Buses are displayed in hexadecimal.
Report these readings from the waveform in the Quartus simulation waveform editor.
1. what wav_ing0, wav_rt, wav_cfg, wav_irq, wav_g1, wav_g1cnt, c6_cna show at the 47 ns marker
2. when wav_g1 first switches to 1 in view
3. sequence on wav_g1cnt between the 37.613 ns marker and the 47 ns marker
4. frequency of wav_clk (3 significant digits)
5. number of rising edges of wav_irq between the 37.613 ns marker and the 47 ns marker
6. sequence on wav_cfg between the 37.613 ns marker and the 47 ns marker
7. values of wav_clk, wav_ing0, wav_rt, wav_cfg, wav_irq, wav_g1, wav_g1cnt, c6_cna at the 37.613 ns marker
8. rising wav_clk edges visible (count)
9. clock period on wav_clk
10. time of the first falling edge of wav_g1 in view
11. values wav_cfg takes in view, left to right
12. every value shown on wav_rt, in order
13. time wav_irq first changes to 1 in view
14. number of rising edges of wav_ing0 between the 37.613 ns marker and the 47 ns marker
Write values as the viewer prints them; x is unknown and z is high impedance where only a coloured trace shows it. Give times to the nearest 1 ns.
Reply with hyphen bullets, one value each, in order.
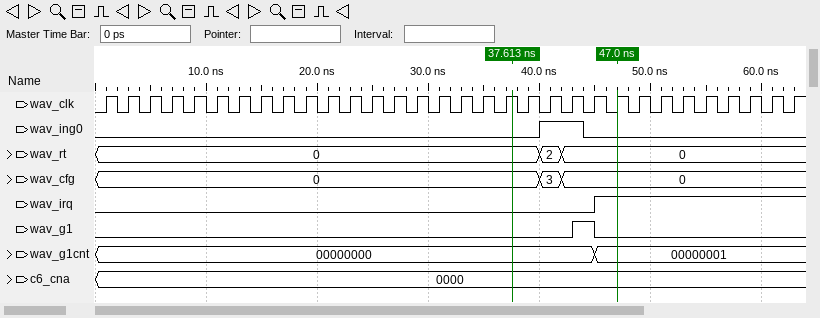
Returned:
- wav_ing0=0, wav_rt=0, wav_cfg=0, wav_irq=1, wav_g1=0, wav_g1cnt=00000001, c6_cna=0000
- 43 ns
- 00000000, 00000001
- 500 MHz
- 1
- 0, 3, 0
- wav_clk=1, wav_ing0=0, wav_rt=0, wav_cfg=0, wav_irq=0, wav_g1=0, wav_g1cnt=00000000, c6_cna=0000
- 32
- 2 ns
- 45 ns
- 0, 3, 0
- 0, 2, 0
- 45 ns
- 1
